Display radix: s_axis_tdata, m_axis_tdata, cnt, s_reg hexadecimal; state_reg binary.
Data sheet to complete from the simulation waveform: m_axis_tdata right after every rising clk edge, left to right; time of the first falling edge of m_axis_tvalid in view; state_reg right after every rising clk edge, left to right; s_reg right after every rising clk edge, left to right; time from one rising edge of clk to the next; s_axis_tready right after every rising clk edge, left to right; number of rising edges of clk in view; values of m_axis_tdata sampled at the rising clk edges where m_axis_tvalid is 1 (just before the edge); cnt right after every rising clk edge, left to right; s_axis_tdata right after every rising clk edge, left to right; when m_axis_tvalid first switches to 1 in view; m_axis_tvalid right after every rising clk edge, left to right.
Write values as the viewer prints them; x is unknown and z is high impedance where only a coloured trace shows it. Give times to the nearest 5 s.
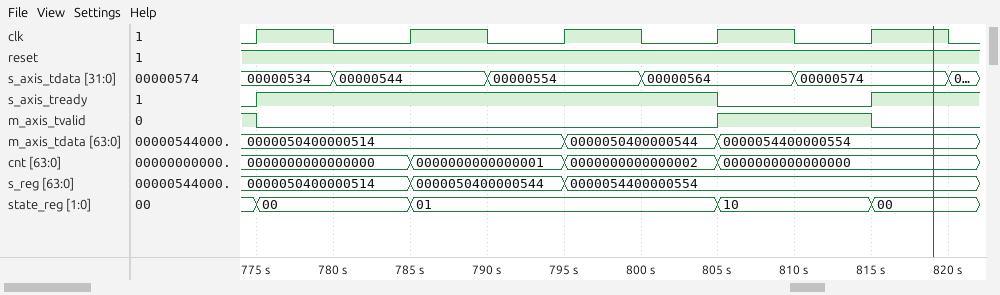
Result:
0000050400000514, 0000050400000514, 0000050400000544, 0000054400000554, 0000054400000554
775 s
00, 01, 01, 10, 00
0000050400000514, 0000050400000544, 0000054400000554, 0000054400000554, 0000054400000554
10 s
1 1 1 0 1
5
0000050400000514, 0000054400000554
0000000000000000, 0000000000000001, 0000000000000002, 0000000000000000, 0000000000000000
00000534, 00000544, 00000554, 00000564, 00000574
805 s
0 0 0 1 0
